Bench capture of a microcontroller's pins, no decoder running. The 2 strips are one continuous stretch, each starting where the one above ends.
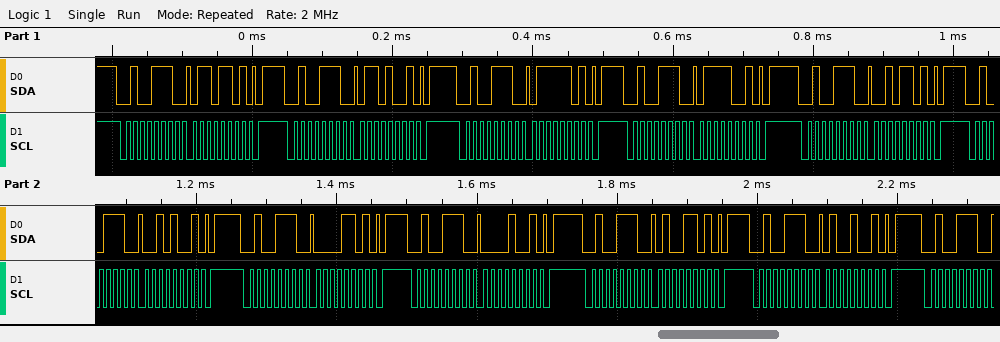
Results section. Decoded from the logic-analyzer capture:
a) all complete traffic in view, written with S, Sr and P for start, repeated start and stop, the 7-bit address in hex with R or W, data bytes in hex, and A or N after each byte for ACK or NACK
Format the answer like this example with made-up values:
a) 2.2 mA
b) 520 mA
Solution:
a) S 27W A 6D A P S 27W A 69 A P S 27W A 7D A P S 27W A 79 A P S 27W A 2D A P S 27W A 29 A P S 27W A 0D A P S 27W A 09 A P S 27W A 4D A P S 27W A 49 A P S 27W A
